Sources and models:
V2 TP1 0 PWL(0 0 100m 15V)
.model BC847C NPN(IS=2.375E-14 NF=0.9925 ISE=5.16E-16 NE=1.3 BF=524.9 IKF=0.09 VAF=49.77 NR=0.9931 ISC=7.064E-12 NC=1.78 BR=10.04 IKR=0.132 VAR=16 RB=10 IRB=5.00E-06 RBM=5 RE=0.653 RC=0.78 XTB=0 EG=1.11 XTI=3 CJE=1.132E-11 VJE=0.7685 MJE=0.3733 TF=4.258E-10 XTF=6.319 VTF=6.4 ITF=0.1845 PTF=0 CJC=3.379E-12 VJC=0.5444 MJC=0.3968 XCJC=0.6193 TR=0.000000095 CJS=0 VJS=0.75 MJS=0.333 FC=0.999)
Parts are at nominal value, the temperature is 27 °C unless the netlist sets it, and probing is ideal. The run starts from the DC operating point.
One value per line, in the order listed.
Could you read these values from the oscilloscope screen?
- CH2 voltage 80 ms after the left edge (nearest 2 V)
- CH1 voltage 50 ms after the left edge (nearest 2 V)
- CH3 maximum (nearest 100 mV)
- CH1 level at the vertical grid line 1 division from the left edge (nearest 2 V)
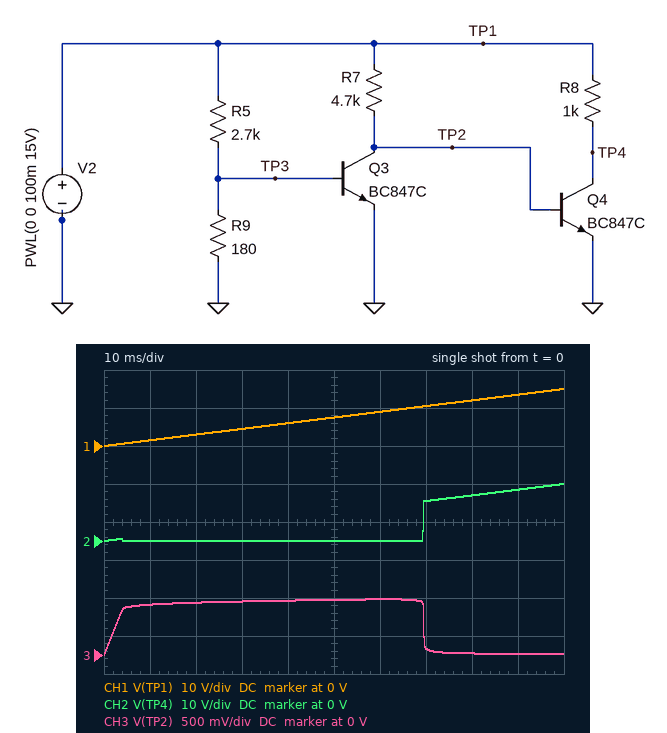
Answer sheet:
12 V
8 V
700 mV
2 V
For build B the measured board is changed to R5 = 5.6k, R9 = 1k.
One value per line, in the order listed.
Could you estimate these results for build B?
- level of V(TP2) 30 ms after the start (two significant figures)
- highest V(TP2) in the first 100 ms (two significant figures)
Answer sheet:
33 mV
690 mV
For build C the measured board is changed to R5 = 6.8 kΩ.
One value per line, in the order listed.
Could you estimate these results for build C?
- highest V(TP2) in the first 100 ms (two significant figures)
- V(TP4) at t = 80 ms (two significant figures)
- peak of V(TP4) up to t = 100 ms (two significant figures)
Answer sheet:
760 mV
36 mV
510 mV
